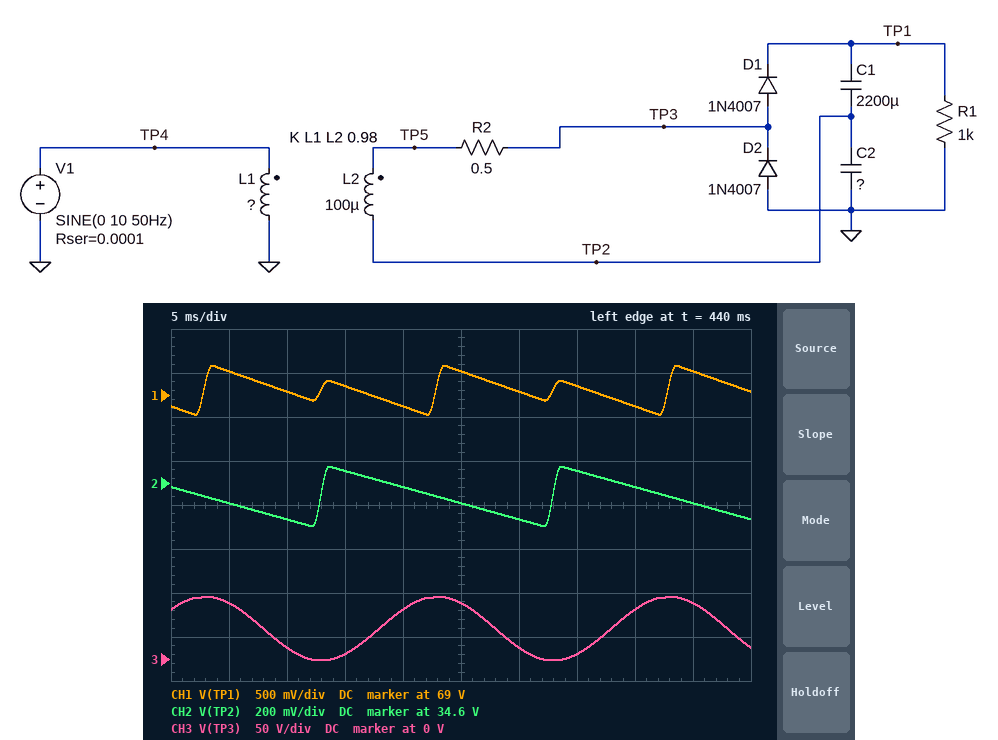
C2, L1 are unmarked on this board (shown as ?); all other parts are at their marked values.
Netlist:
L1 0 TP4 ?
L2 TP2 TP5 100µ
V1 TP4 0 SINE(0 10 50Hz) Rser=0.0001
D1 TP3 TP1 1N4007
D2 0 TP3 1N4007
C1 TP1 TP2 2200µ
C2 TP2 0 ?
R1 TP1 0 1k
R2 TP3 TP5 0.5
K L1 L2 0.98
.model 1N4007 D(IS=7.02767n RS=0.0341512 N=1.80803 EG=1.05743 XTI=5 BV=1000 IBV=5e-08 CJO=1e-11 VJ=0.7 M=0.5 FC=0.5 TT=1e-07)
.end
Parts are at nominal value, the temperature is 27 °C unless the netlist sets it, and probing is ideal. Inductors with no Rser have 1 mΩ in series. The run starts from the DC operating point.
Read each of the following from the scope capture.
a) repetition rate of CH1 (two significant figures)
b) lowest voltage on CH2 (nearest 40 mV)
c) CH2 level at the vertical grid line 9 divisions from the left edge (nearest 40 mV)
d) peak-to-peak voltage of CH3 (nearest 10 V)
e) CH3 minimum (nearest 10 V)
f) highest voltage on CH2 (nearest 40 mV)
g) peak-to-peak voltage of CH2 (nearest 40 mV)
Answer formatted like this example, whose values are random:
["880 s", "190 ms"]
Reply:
["100 Hz", "34.40 V", "34.52 V", "70 V", "0 V", "34.68 V", "280 mV"]
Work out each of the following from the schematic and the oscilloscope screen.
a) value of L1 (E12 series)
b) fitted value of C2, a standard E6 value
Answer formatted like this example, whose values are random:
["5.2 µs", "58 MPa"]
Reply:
["4.7 µH", "4.7 mF"]
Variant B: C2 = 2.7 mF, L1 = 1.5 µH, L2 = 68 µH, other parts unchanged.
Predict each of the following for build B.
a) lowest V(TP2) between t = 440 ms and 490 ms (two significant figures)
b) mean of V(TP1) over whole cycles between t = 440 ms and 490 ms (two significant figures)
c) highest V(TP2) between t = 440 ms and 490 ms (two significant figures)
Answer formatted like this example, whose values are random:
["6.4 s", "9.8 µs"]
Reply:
["24 V", "49 V", "25 V"]
